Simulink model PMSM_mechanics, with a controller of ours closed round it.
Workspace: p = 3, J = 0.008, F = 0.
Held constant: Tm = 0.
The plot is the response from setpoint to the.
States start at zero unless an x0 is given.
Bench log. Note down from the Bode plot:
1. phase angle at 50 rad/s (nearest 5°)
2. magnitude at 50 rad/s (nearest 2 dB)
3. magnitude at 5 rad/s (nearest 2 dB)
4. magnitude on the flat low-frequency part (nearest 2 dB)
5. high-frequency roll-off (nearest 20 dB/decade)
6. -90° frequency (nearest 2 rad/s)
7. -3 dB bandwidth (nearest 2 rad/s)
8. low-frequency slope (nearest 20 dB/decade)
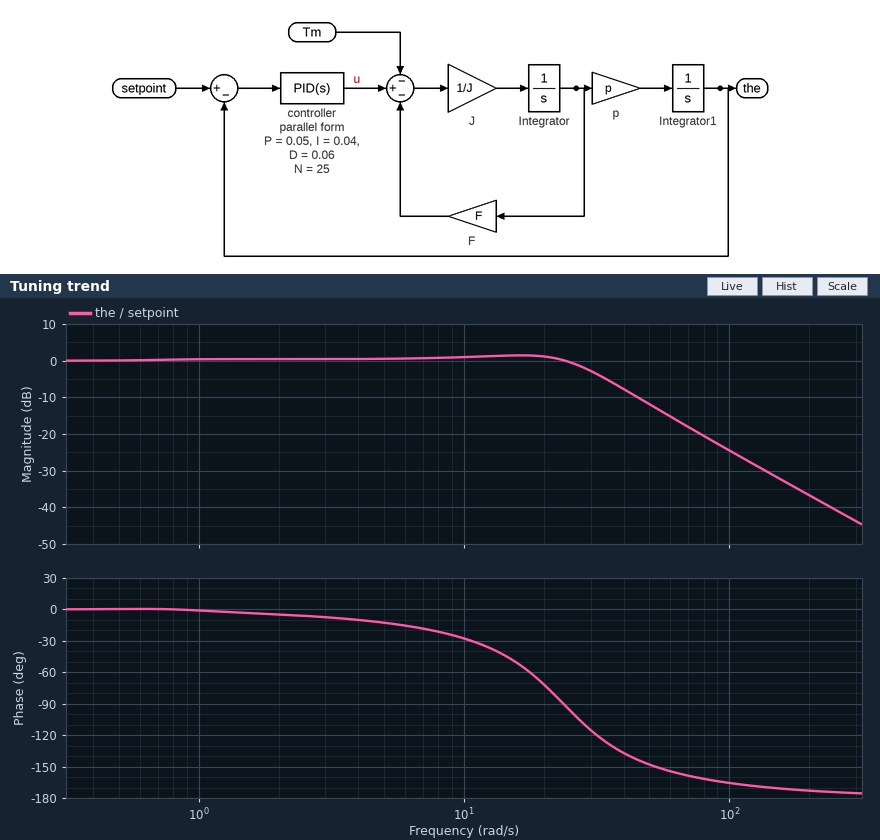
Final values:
-150°
-12 dB
0 dB
0 dB
-40 dB/decade
24 rad/s
30 rad/s
0 dB/decade
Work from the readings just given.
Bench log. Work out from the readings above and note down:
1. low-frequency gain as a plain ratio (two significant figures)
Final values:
1.0
